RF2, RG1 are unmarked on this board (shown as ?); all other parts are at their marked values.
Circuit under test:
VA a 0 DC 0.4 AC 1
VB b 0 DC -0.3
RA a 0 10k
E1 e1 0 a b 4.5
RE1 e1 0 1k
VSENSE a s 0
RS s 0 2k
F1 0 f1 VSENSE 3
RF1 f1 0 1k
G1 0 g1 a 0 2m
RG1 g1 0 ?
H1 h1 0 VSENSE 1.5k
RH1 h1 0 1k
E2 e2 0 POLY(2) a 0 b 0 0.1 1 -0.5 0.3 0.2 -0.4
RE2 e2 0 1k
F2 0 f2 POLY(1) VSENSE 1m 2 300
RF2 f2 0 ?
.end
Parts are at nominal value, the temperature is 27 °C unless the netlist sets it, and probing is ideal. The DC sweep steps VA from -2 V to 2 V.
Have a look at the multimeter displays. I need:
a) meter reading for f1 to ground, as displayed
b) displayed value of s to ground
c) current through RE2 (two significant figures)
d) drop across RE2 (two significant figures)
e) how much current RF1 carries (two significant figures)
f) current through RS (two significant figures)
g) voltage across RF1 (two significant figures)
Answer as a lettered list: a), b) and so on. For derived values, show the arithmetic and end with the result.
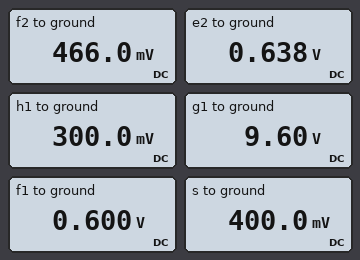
a) 0.600 V
b) 400.0 mV
c) (638 mV) / 1 kΩ = 640 µA
d) 638 mV = 640 mV
e) (600 mV) / 1 kΩ = 600 µA
f) (400 mV) / 2 kΩ = 200 µA
g) 600 mV = 600 mV
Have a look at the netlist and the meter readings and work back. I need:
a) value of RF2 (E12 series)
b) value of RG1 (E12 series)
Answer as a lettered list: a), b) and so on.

a) 330 Ω
b) 12 kΩ
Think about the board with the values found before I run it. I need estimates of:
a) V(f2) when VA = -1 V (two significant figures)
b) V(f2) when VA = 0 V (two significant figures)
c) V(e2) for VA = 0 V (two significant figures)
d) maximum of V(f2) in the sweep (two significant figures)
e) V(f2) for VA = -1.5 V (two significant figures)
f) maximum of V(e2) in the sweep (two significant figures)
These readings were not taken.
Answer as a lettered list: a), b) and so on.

a) 25 mV
b) 330 mV
c) 210 mV
d) 1.1 V
e) -110 mV
f) 3.3 V
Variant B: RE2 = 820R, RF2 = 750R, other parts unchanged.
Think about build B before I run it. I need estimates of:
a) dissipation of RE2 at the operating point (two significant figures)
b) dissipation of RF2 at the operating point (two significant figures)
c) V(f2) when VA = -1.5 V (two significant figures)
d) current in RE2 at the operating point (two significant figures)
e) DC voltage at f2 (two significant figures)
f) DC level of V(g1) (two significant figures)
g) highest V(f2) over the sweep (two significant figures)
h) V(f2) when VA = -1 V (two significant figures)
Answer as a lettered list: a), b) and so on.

a) 500 µW
b) 1.5 mW
c) -250 mV
d) 780 µA
e) 1.1 V
f) 9.6 V
g) 2.5 V
h) 56 mV
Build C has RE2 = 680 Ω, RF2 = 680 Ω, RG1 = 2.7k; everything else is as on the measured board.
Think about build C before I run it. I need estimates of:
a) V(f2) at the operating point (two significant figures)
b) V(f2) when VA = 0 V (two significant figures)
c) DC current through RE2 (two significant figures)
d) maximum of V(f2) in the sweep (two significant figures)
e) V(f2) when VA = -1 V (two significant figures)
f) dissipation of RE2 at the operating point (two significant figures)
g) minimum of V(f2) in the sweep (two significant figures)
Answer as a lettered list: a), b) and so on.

a) 960 mV
b) 680 mV
c) 940 µA
d) 2.2 V
e) 51 mV
f) 600 µW
g) -480 mV
